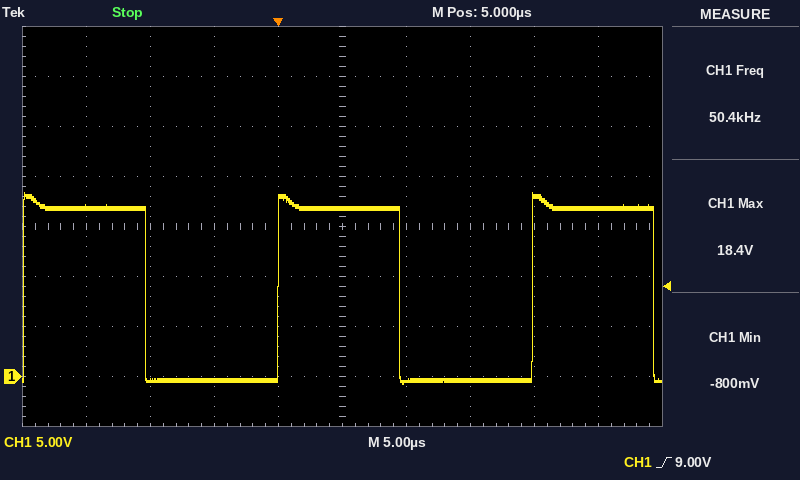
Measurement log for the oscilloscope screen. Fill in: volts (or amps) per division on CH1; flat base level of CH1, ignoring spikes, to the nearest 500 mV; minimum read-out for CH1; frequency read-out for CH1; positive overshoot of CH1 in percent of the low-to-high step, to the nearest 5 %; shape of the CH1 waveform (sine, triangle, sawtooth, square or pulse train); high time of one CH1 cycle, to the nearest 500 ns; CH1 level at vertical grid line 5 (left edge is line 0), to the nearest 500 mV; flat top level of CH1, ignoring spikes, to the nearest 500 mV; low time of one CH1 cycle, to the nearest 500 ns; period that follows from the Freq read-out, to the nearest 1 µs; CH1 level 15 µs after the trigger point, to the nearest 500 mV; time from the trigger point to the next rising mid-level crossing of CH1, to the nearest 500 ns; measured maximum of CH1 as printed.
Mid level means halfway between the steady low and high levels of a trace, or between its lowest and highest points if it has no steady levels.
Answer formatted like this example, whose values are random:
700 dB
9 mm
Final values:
5 V
-500 mV
-800 mV
50.4 kHz
10 %
square
9.5 µs
17.0 V
17.0 V
10.5 µs
20 µs
-500 mV
20.0 µs
18.4 V
